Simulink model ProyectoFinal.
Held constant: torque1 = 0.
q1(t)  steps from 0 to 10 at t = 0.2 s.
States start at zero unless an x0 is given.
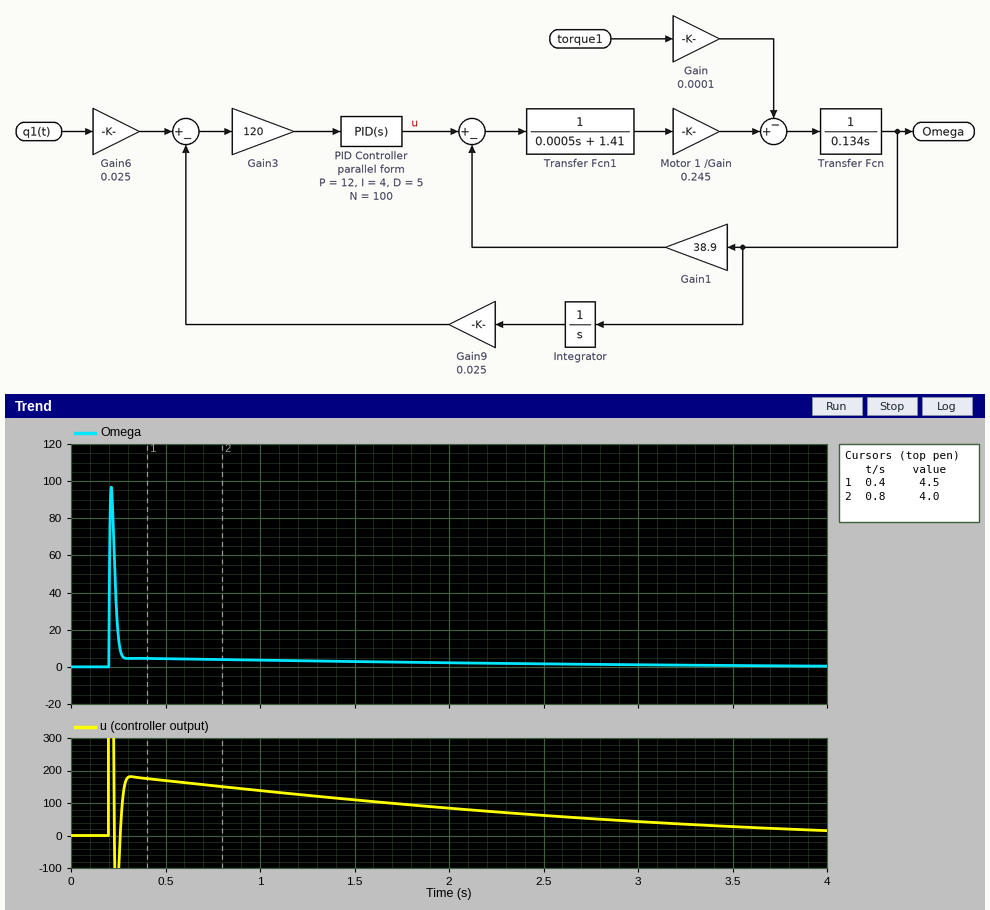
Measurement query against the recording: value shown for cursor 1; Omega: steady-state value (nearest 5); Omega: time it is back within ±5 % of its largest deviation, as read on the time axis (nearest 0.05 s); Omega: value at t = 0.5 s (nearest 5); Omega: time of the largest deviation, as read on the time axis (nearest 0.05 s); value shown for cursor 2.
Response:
4.5
0
0.30 s
5
0.20 s
4.0
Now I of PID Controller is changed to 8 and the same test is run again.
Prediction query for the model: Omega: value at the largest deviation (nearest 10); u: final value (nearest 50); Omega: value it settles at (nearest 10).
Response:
100
0
0
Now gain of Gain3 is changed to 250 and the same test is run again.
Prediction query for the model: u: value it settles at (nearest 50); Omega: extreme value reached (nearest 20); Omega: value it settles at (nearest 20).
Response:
0
200
0
